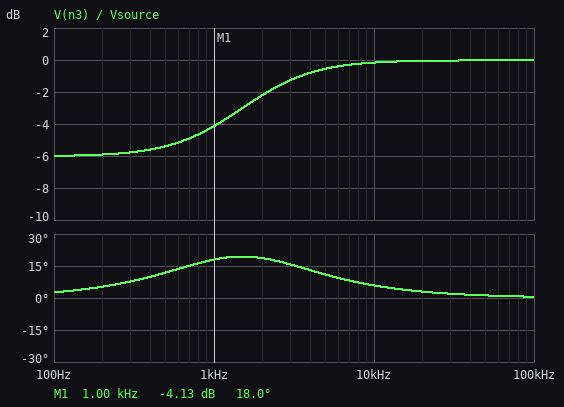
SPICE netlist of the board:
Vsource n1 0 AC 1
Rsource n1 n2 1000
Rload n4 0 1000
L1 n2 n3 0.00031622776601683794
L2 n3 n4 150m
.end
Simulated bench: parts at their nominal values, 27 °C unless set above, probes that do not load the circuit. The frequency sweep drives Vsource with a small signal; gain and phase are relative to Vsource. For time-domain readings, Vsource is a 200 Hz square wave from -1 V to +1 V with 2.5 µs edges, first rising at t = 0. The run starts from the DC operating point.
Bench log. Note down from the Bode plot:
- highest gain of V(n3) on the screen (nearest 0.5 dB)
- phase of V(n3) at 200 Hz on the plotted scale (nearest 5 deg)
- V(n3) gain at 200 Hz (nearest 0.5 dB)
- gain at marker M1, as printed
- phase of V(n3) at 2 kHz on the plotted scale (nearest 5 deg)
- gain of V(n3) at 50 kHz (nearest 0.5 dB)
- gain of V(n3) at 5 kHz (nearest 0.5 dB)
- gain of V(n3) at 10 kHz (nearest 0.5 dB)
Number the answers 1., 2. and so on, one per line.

1. 0 dB
2. 5 deg
3. -6.0 dB
4. -4.13 dB
5. 20 deg
6. 0 dB
7. -0.5 dB
8. 0 dB
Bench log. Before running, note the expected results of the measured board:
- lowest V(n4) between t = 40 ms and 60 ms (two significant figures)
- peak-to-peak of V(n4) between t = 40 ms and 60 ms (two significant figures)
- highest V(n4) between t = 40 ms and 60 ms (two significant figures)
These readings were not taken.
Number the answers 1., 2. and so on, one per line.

1. -500 mV
2. 1.0 V
3. 500 mV
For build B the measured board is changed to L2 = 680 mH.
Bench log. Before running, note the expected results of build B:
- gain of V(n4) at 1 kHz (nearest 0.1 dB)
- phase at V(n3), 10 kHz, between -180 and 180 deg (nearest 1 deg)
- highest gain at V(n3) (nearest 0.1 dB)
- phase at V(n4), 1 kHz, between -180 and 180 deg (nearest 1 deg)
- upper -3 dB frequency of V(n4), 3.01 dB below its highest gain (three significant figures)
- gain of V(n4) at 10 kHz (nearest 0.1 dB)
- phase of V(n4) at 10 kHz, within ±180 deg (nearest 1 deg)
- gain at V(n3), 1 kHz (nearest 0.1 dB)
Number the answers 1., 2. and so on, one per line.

1. -13.5 dB
2. 1 deg
3. 0 dB
4. -65 deg
5. 468 Hz
6. -32.6 dB
7. -87 deg
8. -0.6 dB
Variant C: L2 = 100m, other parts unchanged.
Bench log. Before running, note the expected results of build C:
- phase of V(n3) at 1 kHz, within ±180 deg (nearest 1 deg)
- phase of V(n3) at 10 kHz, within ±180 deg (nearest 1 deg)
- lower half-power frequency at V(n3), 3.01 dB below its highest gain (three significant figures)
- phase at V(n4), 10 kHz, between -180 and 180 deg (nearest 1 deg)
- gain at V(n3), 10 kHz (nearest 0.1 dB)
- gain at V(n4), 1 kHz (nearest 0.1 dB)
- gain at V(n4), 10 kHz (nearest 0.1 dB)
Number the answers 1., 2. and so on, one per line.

1. 15 deg
2. 9 deg
3. 2.24 kHz
4. -72 deg
5. -0.3 dB
6. -6.4 dB
7. -16.4 dB
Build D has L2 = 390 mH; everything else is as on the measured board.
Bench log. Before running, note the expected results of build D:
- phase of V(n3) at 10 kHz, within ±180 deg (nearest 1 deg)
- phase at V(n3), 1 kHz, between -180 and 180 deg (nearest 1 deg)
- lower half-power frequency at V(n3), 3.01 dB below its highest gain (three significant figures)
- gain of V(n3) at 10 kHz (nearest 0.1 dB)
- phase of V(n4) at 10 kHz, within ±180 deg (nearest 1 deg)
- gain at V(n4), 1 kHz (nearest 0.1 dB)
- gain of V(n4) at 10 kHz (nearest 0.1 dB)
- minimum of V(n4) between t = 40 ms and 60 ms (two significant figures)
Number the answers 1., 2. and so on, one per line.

1. 2 deg
2. 17 deg
3. 576 Hz
4. 0 dB
5. -85 deg
6. -10.0 dB
7. -27.8 dB
8. -500 mV
